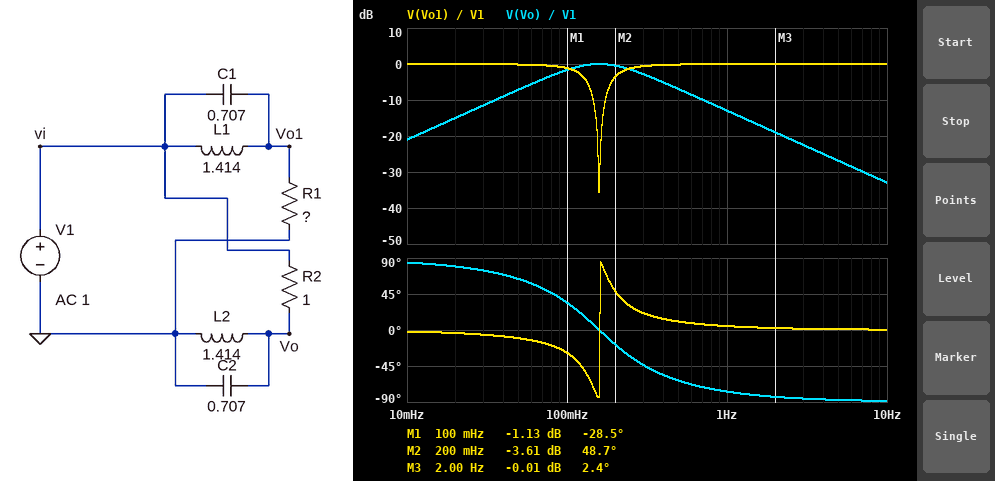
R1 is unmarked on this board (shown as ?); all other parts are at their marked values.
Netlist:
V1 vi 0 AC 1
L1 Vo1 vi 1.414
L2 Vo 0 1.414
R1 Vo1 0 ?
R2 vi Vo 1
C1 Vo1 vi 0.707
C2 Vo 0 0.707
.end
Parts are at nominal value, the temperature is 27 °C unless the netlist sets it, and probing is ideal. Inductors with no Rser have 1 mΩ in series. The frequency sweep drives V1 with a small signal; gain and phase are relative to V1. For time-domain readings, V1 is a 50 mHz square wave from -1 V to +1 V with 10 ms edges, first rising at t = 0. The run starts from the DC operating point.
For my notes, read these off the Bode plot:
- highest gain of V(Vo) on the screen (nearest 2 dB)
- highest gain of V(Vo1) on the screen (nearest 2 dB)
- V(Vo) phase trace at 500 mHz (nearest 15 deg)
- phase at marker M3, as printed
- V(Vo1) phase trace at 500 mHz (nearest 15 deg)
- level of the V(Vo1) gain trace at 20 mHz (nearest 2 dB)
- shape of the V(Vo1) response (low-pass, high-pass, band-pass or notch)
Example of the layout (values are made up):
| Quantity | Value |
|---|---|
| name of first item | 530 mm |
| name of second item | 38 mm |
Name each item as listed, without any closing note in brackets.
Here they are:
| Quantity | Value |
|---|---|
| highest gain of V(Vo) on the screen | 0 dB |
| highest gain of V(Vo1) on the screen | 0 dB |
| V(Vo) phase trace at 500 mHz | -60 deg |
| phase at marker M3, as printed | 2.4 deg |
| V(Vo1) phase trace at 500 mHz | 15 deg |
| level of the V(Vo1) gain trace at 20 mHz | 0 dB |
| shape of the V(Vo1) response | notch |
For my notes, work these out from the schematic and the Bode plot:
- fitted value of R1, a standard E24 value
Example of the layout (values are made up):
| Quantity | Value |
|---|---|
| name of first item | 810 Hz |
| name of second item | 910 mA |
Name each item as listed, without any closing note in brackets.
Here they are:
| Quantity | Value |
|---|---|
| fitted value of R1, a standard E24 value | 2.7 Ω |
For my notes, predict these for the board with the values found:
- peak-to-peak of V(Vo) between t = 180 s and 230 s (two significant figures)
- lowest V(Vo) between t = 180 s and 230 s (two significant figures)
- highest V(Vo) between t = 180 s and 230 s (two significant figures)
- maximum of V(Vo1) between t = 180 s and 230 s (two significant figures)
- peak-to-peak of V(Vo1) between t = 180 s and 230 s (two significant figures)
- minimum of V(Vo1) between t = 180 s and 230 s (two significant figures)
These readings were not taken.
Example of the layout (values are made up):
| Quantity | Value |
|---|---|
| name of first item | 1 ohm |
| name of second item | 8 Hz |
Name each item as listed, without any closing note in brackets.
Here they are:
| Quantity | Value |
|---|---|
| peak-to-peak of V(Vo) between t = 180 s and 230 s | 2.6 V |
| lowest V(Vo) between t = 180 s and 230 s | -1.3 V |
| highest V(Vo) between t = 180 s and 230 s | 1.3 V |
| maximum of V(Vo1) between t = 180 s and 230 s | 1.3 V |
| peak-to-peak of V(Vo1) between t = 180 s and 230 s | 2.7 V |
| minimum of V(Vo1) between t = 180 s and 230 s | -1.3 V |
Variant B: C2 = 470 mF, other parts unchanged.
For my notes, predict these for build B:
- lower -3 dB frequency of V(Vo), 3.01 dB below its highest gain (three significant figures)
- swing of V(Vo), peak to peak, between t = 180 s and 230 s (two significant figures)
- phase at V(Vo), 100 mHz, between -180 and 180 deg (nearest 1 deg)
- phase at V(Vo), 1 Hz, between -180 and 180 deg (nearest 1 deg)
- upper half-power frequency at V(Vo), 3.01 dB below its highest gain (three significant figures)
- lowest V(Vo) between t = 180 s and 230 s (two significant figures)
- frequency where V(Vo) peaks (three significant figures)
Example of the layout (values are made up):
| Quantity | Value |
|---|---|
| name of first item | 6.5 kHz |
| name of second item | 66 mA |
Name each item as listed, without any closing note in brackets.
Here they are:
| Quantity | Value |
|---|---|
| lower -3 dB frequency of V(Vo), 3.01 dB below its highest gain | 89.2 mHz |
| swing of V(Vo), peak to peak, between t = 180 s and 230 s | 2.8 V |
| phase at V(Vo), 100 mHz, between -180 and 180 deg | 40 deg |
| phase at V(Vo), 1 Hz, between -180 and 180 deg | -71 deg |
| upper half-power frequency at V(Vo), 3.01 dB below its highest gain | 428 mHz |
| lowest V(Vo) between t = 180 s and 230 s | -1.4 V |
| frequency where V(Vo) peaks | 195 mHz |
